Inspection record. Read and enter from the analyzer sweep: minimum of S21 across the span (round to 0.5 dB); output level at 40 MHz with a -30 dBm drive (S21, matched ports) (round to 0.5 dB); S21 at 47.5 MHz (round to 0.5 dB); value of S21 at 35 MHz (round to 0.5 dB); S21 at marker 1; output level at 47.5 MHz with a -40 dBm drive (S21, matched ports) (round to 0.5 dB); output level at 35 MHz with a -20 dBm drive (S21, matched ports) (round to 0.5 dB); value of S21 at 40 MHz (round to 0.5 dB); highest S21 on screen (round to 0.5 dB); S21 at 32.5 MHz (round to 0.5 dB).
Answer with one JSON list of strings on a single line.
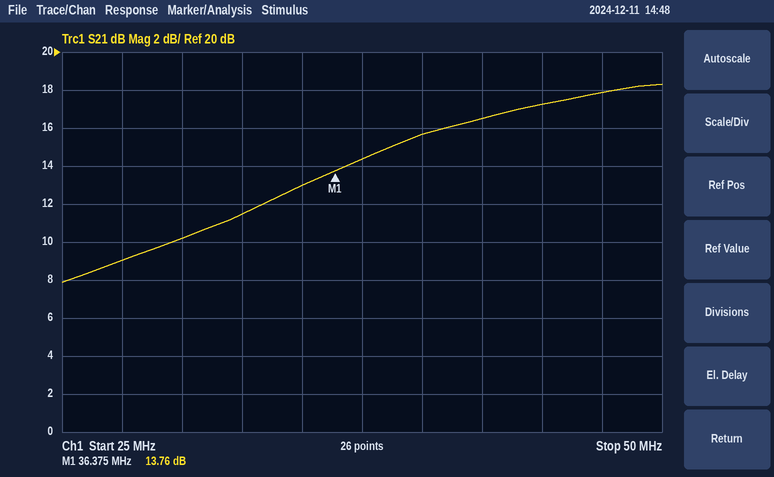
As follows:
["8.0 dB", "-14.5 dBm", "18.0 dB", "13.0 dB", "13.76 dB", "-22.0 dBm", "-7.0 dBm", "15.5 dB", "18.5 dB", "11.5 dB"]
